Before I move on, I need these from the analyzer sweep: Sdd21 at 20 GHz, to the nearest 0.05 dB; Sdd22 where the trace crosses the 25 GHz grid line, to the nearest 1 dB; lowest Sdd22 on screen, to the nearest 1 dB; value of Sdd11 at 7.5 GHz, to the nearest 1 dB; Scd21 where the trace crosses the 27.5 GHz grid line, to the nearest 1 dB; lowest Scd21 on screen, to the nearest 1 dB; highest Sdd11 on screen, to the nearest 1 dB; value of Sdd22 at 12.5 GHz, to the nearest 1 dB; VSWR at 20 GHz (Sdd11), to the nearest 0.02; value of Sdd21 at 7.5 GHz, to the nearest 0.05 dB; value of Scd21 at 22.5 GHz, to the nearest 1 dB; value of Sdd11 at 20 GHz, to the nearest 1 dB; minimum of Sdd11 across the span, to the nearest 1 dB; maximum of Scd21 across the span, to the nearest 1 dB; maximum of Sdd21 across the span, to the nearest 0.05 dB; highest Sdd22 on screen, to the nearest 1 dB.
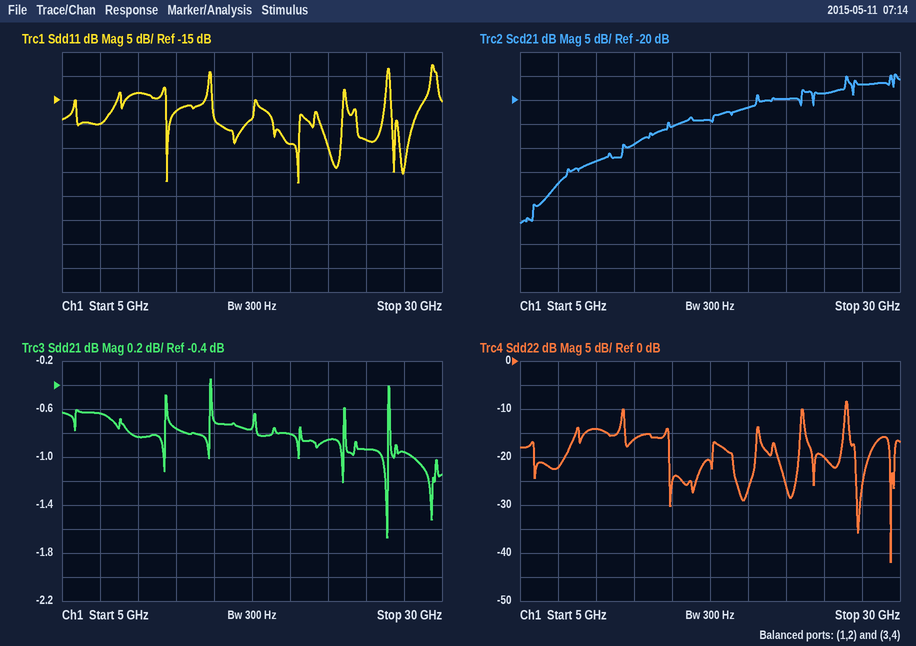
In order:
-0.80 dB
-20 dB
-42 dB
-20 dB
-17 dB
-46 dB
-8 dB
-16 dB
1.14
-0.65 dB
-20 dB
-24 dB
-32 dB
-15 dB
-0.35 dB
-8 dB
